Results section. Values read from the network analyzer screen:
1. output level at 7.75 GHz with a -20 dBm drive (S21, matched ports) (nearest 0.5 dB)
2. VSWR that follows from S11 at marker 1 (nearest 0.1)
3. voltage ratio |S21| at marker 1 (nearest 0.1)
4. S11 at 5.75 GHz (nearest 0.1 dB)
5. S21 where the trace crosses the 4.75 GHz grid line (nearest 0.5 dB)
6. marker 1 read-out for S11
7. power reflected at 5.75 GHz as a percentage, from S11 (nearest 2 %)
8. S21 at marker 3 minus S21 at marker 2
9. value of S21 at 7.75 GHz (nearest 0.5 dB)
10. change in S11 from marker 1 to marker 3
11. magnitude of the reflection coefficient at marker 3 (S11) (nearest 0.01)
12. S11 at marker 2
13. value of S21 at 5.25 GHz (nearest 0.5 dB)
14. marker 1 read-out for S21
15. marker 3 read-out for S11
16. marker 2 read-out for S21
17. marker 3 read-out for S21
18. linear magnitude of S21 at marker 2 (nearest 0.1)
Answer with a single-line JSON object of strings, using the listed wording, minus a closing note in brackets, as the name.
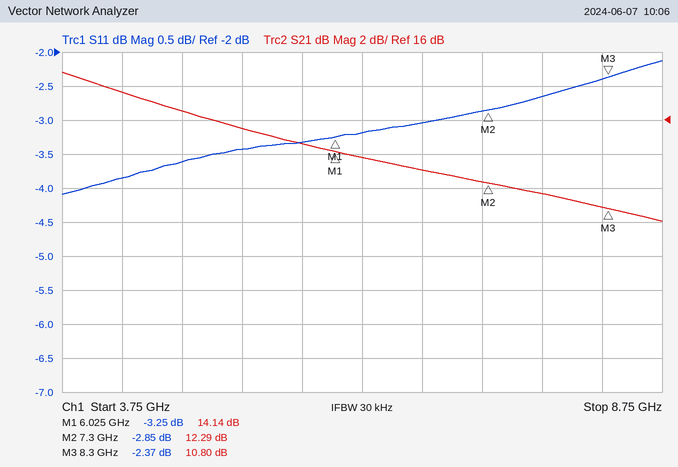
{"output level at 7.75 GHz with a -20 dBm drive (S21, matched ports)": "-8.5 dBm", "VSWR that follows from S11 at marker 1": "5.4", "voltage ratio |S21| at marker 1": "5.1", "S11 at 5.75 GHz": "-3.3 dB", "S21 where the trace crosses the 4.75 GHz grid line": "16.5 dB", "marker 1 read-out for S11": "-3.25 dB", "power reflected at 5.75 GHz as a percentage, from S11": "46 %", "S21 at marker 3 minus S21 at marker 2": "-1.49 dB", "value of S21 at 7.75 GHz": "11.5 dB", "change in S11 from marker 1 to marker 3": "0.88 dB", "magnitude of the reflection coefficient at marker 3 (S11)": "0.76", "S11 at marker 2": "-2.85 dB", "value of S21 at 5.25 GHz": "15.5 dB", "marker 1 read-out for S21": "14.14 dB", "marker 3 read-out for S11": "-2.37 dB", "marker 2 read-out for S21": "12.29 dB", "marker 3 read-out for S21": "10.80 dB", "linear magnitude of S21 at marker 2": "4.1"}
